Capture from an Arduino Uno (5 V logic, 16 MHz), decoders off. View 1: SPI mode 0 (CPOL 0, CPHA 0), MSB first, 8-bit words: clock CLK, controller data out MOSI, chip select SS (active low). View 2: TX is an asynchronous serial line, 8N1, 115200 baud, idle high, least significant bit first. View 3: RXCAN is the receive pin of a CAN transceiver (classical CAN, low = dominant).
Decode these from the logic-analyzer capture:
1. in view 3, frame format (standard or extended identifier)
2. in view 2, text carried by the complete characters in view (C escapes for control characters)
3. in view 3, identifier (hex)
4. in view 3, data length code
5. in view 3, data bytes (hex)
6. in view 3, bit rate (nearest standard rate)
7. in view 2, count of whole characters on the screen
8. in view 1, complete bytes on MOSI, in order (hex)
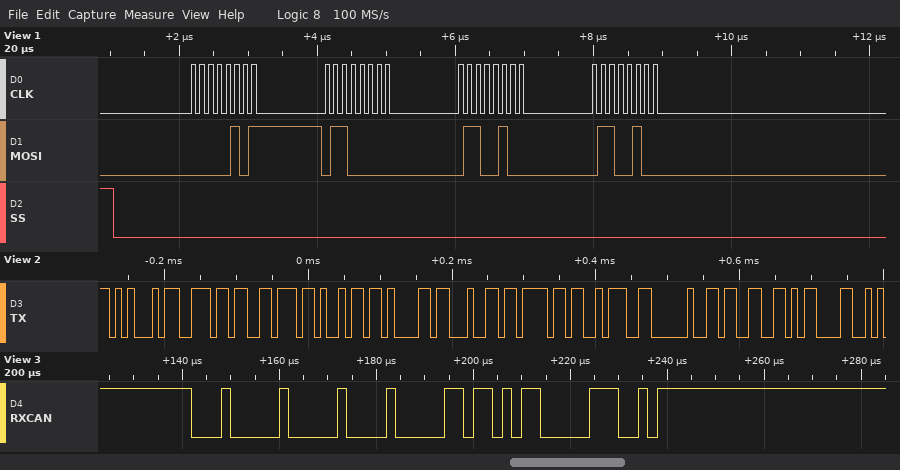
standard
"Enviado: 3\r"
0x100
1
05
500 kbit/s
11
05 60 64 64
